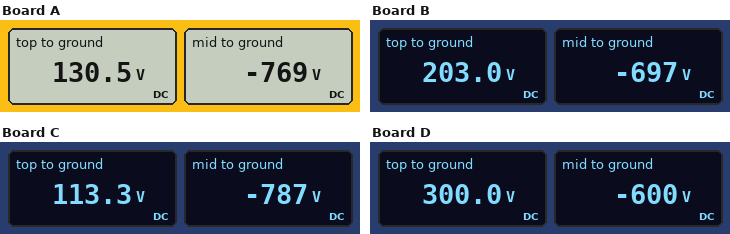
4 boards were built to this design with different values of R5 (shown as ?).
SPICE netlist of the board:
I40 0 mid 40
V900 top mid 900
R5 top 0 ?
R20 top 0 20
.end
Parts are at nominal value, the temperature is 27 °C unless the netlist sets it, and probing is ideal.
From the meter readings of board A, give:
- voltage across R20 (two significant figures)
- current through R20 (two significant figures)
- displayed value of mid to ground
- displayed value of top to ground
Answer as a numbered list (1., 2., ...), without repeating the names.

1. 130 V
2. 6.5 A
3. -769 V
4. 130.5 V
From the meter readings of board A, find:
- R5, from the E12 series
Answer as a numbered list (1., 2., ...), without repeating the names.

1. 3.9 Ω
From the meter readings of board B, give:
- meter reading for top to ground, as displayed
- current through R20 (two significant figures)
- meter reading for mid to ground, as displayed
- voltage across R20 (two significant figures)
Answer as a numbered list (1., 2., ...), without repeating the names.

1. 203.0 V
2. 10 A
3. -697 V
4. 200 V
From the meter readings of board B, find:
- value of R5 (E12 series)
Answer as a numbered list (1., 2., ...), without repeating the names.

1. 6.8 Ω
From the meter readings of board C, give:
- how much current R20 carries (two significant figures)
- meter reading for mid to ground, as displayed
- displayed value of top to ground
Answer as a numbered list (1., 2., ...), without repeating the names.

1. 5.7 A
2. -787 V
3. 113.3 V
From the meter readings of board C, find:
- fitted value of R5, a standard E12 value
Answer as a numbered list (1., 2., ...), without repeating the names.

1. 3.3 Ω
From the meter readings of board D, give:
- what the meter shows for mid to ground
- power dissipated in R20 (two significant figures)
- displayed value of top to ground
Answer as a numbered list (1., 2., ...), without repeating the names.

1. -600 V
2. 4.5 kW
3. 300.0 V
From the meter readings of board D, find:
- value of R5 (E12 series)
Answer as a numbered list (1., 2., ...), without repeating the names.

1. 12 Ω
